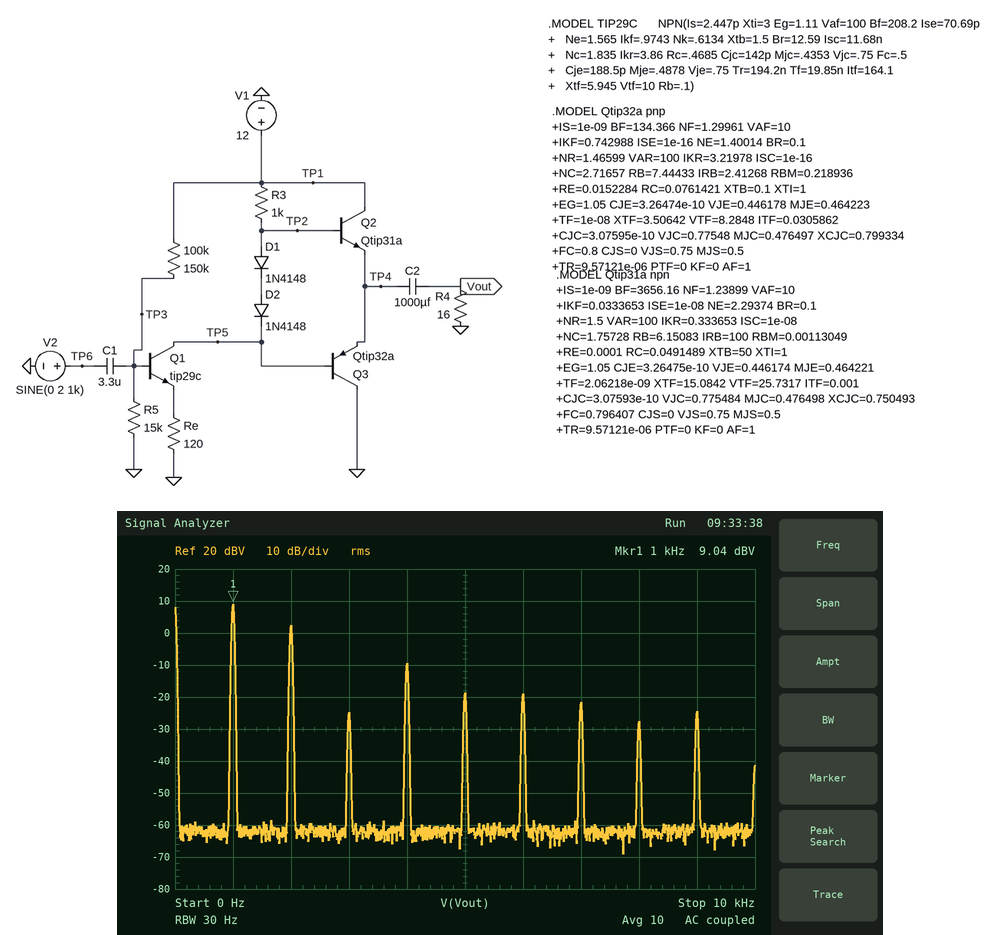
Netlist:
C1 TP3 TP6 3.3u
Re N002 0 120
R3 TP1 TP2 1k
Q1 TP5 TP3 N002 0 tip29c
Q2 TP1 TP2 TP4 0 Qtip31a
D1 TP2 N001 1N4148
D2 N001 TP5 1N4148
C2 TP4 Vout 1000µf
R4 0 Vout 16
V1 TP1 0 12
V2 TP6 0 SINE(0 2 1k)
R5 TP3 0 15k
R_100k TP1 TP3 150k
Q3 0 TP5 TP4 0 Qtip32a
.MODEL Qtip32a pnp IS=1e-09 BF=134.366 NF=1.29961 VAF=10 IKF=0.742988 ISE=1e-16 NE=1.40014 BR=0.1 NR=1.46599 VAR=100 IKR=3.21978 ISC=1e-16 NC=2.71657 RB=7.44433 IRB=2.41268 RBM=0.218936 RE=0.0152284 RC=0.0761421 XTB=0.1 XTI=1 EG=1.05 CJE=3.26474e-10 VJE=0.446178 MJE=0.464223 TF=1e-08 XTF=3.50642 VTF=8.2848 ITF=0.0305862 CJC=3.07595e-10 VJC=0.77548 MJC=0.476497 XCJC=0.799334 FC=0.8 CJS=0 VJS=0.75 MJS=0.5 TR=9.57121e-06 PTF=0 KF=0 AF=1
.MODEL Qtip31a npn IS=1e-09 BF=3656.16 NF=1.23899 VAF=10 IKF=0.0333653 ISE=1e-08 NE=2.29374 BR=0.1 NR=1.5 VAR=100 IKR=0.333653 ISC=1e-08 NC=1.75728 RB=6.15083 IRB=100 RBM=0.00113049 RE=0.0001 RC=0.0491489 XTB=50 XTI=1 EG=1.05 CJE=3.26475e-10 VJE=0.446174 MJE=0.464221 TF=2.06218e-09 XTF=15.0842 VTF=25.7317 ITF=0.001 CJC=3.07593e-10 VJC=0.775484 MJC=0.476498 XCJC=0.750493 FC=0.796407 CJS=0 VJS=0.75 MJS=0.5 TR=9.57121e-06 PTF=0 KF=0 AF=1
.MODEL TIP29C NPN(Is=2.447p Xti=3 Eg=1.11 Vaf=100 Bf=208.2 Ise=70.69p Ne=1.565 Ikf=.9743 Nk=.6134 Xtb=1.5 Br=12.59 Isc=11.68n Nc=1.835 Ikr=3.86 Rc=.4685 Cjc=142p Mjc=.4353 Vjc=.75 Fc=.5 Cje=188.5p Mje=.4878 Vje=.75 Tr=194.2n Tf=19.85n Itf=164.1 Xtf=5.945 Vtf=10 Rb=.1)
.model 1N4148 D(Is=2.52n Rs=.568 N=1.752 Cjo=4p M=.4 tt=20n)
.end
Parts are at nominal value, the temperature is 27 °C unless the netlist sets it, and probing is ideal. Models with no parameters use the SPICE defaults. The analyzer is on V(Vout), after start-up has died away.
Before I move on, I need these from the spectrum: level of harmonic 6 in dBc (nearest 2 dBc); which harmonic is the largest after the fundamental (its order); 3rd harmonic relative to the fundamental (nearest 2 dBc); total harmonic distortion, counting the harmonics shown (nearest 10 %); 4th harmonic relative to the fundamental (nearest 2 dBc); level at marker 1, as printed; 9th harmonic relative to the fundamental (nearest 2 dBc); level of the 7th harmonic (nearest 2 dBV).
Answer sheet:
-28 dBc
2
-34 dBc
50 %
-18 dBc
9.04 dBV
-34 dBc
-22 dBV
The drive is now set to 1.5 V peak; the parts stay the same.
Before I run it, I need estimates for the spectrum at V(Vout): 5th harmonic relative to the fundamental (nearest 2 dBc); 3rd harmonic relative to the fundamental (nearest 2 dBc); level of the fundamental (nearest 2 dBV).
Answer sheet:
-34 dBc
-56 dBc
8 dBV
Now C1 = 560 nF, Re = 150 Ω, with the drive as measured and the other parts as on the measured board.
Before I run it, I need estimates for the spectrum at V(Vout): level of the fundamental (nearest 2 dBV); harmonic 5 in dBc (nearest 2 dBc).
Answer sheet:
8 dBV
-34 dBc
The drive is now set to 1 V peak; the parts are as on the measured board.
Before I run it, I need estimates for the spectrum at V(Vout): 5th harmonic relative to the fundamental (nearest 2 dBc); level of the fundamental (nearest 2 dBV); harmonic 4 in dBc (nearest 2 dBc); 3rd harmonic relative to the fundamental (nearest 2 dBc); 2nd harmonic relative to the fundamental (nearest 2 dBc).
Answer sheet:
-46 dBc
6 dBV
-20 dBc
-30 dBc
-8 dBc
